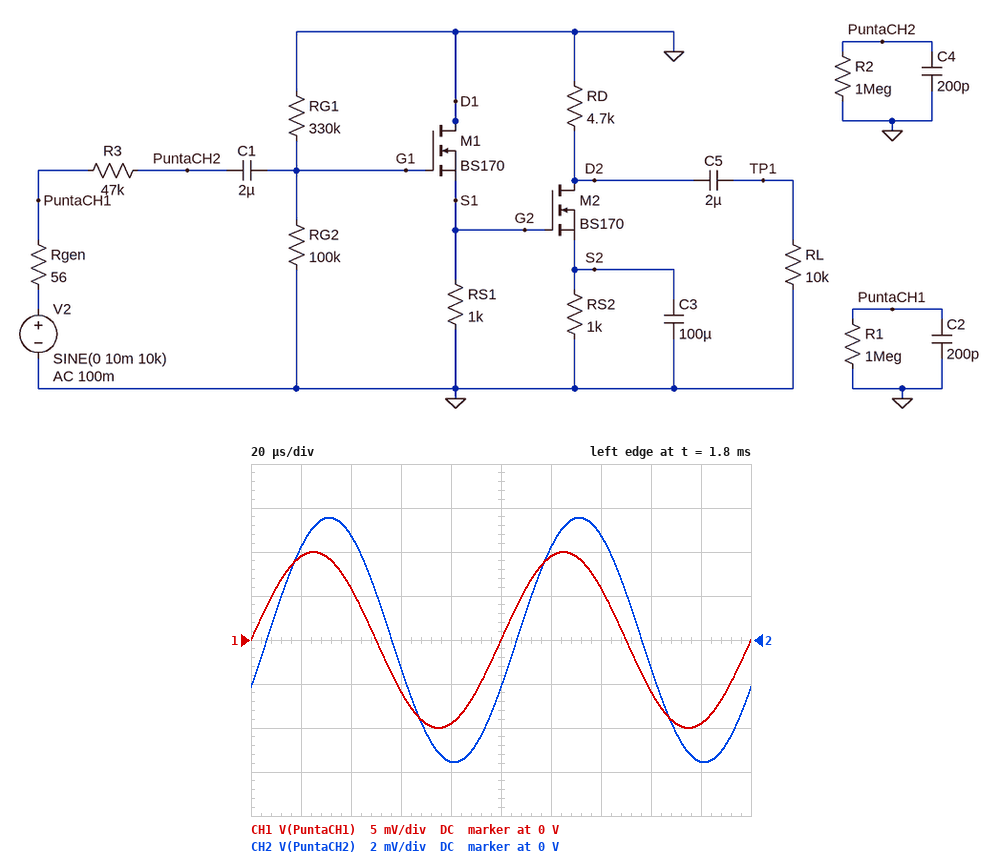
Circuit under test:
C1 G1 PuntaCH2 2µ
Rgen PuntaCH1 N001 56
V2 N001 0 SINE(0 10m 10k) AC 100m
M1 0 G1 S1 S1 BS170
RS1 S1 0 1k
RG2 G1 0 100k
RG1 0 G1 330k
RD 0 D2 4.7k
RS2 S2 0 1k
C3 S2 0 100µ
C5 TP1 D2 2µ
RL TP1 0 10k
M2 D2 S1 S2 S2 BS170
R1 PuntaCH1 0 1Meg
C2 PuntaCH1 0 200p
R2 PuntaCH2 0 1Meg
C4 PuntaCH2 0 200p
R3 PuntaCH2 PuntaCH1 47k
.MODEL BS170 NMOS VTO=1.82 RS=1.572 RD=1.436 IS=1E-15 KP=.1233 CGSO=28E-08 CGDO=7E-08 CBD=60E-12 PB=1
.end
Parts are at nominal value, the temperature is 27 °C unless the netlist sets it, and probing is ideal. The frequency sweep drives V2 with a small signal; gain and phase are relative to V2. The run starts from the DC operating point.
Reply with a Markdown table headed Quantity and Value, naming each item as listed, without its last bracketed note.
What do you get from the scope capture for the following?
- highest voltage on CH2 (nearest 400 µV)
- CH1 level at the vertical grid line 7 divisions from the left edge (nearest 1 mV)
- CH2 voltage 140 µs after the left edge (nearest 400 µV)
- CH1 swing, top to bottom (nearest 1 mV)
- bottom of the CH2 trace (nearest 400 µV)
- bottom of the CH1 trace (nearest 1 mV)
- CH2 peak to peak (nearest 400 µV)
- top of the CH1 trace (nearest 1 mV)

| Quantity | Value |
|---|---|
| highest voltage on CH2 | 5.6 mV |
| CH1 level at the vertical grid line 7 divisions from the left edge | 6 mV |
| CH2 voltage 140 µs after the left edge | 4.8 mV |
| CH1 swing, top to bottom | 20 mV |
| bottom of the CH2 trace | -5.6 mV |
| bottom of the CH1 trace | -10 mV |
| CH2 peak to peak | 11.2 mV |
| top of the CH1 trace | 10 mV |
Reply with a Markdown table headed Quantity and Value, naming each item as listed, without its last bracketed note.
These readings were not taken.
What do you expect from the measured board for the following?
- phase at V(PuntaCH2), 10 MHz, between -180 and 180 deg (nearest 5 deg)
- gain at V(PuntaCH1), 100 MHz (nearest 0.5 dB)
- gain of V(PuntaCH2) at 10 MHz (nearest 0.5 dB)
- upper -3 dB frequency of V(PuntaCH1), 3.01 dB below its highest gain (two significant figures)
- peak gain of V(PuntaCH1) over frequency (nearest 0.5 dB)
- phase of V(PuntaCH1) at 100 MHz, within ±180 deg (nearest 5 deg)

| Quantity | Value |
|---|---|
| phase at V(PuntaCH2), 10 MHz, between -180 and 180 deg | -125 deg |
| gain at V(PuntaCH1), 100 MHz | -17.0 dB |
| gain of V(PuntaCH2) at 10 MHz | -58.5 dB |
| upper -3 dB frequency of V(PuntaCH1), 3.01 dB below its highest gain | 14 MHz |
| peak gain of V(PuntaCH1) over frequency | 0 dB |
| phase of V(PuntaCH1) at 100 MHz, within ±180 deg | -80 deg |
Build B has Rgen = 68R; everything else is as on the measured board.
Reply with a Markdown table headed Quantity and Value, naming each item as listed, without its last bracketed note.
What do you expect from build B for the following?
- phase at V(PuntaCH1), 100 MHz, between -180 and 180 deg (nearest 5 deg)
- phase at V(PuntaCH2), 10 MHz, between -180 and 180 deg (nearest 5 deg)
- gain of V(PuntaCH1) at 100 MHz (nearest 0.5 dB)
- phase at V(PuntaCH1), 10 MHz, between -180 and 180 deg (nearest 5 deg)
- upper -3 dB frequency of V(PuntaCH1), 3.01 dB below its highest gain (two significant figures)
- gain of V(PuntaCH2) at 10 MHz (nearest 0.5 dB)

| Quantity | Value |
|---|---|
| phase at V(PuntaCH1), 100 MHz, between -180 and 180 deg | -85 deg |
| phase at V(PuntaCH2), 10 MHz, between -180 and 180 deg | -130 deg |
| gain of V(PuntaCH1) at 100 MHz | -18.5 dB |
| phase at V(PuntaCH1), 10 MHz, between -180 and 180 deg | -40 deg |
| upper -3 dB frequency of V(PuntaCH1), 3.01 dB below its highest gain | 12 MHz |
| gain of V(PuntaCH2) at 10 MHz | -59.0 dB |
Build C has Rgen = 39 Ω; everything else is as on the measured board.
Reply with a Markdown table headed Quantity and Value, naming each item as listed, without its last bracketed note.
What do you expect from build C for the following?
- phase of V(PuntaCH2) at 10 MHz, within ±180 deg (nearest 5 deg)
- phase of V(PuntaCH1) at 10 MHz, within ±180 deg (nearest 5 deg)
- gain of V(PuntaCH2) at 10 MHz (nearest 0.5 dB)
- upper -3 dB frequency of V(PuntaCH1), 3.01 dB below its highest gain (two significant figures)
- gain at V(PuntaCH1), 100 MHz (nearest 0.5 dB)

| Quantity | Value |
|---|---|
| phase of V(PuntaCH2) at 10 MHz, within ±180 deg | -115 deg |
| phase of V(PuntaCH1) at 10 MHz, within ±180 deg | -25 deg |
| gain of V(PuntaCH2) at 10 MHz | -57.5 dB |
| upper -3 dB frequency of V(PuntaCH1), 3.01 dB below its highest gain | 20 MHz |
| gain at V(PuntaCH1), 100 MHz | -14.0 dB |
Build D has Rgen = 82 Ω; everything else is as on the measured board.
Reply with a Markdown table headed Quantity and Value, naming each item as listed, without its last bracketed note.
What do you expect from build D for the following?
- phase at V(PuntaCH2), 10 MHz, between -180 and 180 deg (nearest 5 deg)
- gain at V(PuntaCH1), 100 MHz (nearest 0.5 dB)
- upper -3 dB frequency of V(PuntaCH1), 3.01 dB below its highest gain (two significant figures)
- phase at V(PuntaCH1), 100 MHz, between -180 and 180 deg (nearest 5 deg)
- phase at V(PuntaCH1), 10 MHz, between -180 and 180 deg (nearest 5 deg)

| Quantity | Value |
|---|---|
| phase at V(PuntaCH2), 10 MHz, between -180 and 180 deg | -135 deg |
| gain at V(PuntaCH1), 100 MHz | -20.5 dB |
| upper -3 dB frequency of V(PuntaCH1), 3.01 dB below its highest gain | 9.7 MHz |
| phase at V(PuntaCH1), 100 MHz, between -180 and 180 deg | -85 deg |
| phase at V(PuntaCH1), 10 MHz, between -180 and 180 deg | -45 deg |
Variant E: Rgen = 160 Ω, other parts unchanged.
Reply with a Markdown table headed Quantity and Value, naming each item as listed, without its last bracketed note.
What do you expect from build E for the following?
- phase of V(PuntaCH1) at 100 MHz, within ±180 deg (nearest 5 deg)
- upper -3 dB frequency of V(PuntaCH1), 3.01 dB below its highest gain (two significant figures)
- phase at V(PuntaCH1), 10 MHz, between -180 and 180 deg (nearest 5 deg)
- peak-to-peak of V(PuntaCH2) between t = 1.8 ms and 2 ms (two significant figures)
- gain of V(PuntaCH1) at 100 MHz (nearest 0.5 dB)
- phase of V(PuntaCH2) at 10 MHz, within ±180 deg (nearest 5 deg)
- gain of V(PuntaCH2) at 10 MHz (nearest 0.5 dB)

| Quantity | Value |
|---|---|
| phase of V(PuntaCH1) at 100 MHz, within ±180 deg | -85 deg |
| upper -3 dB frequency of V(PuntaCH1), 3.01 dB below its highest gain | 5.0 MHz |
| phase at V(PuntaCH1), 10 MHz, between -180 and 180 deg | -65 deg |
| peak-to-peak of V(PuntaCH2) between t = 1.8 ms and 2 ms | 11 mV |
| gain of V(PuntaCH1) at 100 MHz | -26.0 dB |
| phase of V(PuntaCH2) at 10 MHz, within ±180 deg | -155 deg |
| gain of V(PuntaCH2) at 10 MHz | -63.5 dB |
